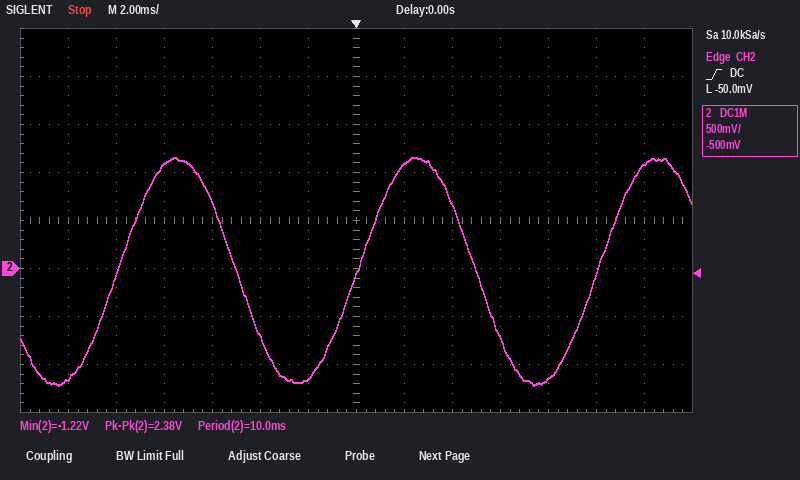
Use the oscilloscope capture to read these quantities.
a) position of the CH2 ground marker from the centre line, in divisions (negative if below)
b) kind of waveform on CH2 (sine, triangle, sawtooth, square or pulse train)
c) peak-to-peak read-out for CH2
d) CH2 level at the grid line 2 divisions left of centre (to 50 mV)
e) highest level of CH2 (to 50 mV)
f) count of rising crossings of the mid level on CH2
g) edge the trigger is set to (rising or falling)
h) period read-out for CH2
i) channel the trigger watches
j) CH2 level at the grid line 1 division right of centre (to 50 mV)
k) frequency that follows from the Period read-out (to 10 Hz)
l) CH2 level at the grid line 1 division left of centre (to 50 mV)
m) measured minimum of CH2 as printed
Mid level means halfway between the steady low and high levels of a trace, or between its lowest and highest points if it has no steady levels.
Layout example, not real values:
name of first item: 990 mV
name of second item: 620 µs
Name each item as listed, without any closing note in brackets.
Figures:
position of the CH2 ground marker from the centre line, in divisions: -1.0 div
kind of waveform on CH2: sine
peak-to-peak read-out for CH2: 2.38 V
CH2 level at the grid line 2 divisions left of centre: -700 mV
highest level of CH2: 1.15 V
count of rising crossings of the mid level on CH2: 3
edge the trigger is set to: rising
period read-out for CH2: 10.0 ms
channel the trigger watches: CH2
CH2 level at the grid line 1 division right of centre: 1.10 V
frequency that follows from the Period read-out: 100 Hz
CH2 level at the grid line 1 division left of centre: -1.15 V
measured minimum of CH2 as printed: -1.22 V
